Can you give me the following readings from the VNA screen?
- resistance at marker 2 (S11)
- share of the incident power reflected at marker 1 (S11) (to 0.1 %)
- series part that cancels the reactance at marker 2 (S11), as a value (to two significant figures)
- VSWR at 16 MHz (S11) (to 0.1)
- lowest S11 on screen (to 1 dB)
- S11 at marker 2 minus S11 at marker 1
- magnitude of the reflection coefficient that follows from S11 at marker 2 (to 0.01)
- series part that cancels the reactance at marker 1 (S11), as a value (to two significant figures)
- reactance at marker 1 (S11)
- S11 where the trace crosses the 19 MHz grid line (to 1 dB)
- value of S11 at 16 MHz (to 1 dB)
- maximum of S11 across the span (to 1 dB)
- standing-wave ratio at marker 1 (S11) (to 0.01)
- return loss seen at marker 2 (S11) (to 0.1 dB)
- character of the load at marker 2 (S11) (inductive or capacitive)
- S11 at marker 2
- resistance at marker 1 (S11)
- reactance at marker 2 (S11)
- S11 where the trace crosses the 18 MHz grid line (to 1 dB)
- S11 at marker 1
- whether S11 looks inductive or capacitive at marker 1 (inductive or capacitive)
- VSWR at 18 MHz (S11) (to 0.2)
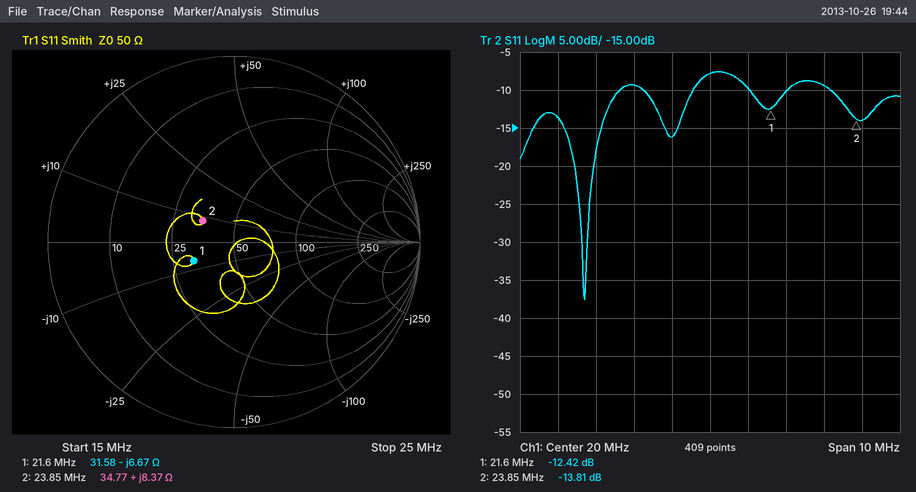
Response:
34.77 Ω
5.7 %
800 pF
1.5
-38 dB
-1.39 dB
0.20
49 nH
-6.67 Ω
-16 dB
-14 dB
-8 dB
1.63
13.8 dB
inductive
-13.81 dB
31.58 Ω
+8.37 Ω
-9 dB
-12.42 dB
capacitive
2.0
